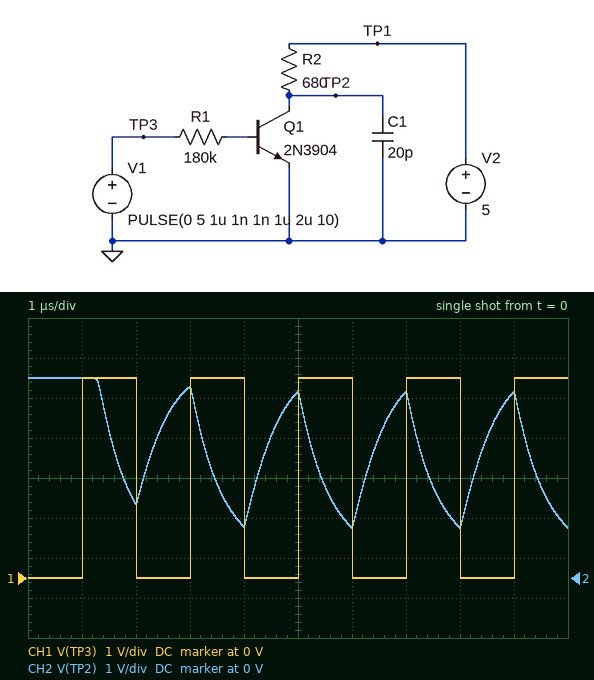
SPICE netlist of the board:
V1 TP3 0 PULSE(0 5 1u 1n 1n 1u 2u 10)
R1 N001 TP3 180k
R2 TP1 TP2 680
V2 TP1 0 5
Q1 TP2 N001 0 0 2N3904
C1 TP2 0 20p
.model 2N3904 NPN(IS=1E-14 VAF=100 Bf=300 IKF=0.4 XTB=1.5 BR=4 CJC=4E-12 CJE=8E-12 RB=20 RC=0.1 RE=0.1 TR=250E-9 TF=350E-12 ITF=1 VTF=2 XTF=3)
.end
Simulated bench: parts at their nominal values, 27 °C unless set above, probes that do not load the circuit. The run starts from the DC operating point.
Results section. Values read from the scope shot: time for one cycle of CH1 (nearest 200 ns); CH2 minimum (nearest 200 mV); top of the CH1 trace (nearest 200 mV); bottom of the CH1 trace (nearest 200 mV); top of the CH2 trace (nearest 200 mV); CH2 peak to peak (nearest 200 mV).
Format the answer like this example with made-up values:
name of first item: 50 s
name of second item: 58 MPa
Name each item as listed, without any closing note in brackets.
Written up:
time for one cycle of CH1: 2.0 µs
CH2 minimum: 1.2 V
top of the CH1 trace: 5.0 V
bottom of the CH1 trace: 0 V
top of the CH2 trace: 5.0 V
CH2 peak to peak: 3.8 V
